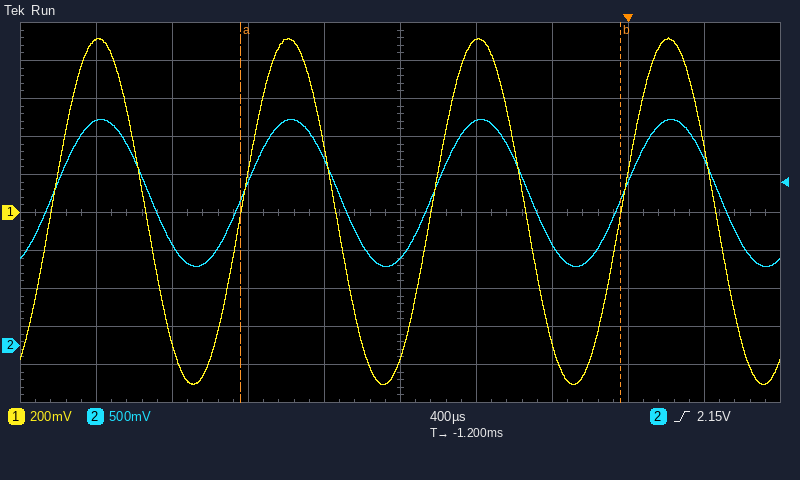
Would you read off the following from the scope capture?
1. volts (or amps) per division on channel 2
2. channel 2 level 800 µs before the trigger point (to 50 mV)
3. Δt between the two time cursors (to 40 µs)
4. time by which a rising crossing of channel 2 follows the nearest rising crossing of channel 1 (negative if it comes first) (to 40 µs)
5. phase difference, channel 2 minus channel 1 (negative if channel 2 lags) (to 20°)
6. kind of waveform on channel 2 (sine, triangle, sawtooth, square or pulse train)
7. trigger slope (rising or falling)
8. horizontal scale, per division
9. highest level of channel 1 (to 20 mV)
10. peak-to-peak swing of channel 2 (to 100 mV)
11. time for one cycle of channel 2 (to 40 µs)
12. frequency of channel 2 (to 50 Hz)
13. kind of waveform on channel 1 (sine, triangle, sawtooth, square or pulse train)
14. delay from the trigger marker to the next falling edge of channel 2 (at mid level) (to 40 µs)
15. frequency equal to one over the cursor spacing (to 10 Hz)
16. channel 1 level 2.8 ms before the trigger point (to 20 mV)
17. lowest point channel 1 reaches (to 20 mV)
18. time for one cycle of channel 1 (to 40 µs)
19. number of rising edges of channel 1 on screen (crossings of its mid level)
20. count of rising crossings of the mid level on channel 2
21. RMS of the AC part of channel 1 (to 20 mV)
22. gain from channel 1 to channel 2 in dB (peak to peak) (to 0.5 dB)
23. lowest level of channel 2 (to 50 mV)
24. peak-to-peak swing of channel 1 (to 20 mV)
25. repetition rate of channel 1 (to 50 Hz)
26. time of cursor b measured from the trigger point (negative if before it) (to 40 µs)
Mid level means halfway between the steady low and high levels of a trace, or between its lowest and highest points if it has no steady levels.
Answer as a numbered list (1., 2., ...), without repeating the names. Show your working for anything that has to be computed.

1. 500 mV
2. 2.95 V
3. 2.00 ms
4. 0 µs
5. −360° × (0 µs) / 1.00 ms ≈ 0°
6. sine
7. rising
8. 400 µs
9. 920 mV
10. 1.90 V
11. 1.00 ms
12. 1 / 1.00 ms ≈ 1.00 kHz
13. sine
14. 480 µs
15. 1 / 2.00 ms ≈ 500 Hz
16. 900 mV
17. -900 mV
18. 1.00 ms
19. 4
20. 4
21. 1.82 V / (2√2) ≈ 643 mV, so 640 mV to the nearest 20 mV
22. 20 log10(1.90 V / 1.82 V) ≈ 0.374 dB, so 0.5 dB to the nearest 0.5 dB
23. 1.05 V
24. 920 mV − (-900 mV) = 1.82 V
25. 1 / 1.00 ms ≈ 1.00 kHz
26. -40 µs
